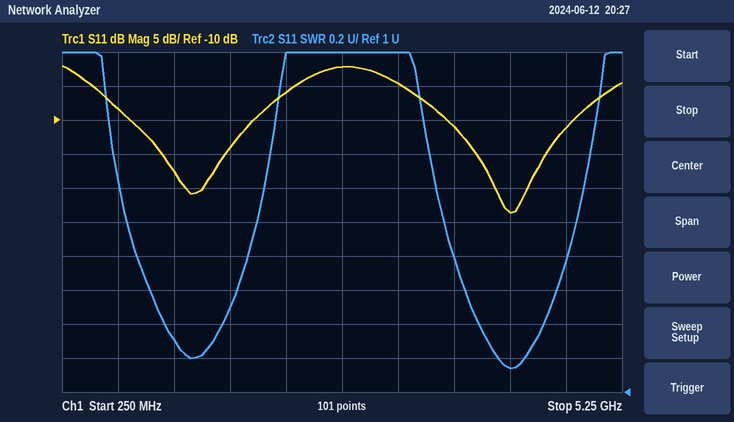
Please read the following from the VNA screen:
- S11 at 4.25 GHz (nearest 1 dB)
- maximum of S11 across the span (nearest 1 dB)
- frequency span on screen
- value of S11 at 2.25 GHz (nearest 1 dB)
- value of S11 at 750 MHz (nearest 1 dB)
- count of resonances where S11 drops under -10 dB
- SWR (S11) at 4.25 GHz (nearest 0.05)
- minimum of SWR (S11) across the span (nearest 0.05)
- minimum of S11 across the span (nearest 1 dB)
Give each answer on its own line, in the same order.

-24 dB
-2 dB
5 GHz
-6 dB
-8 dB
2
1.15
1.15
-24 dB
